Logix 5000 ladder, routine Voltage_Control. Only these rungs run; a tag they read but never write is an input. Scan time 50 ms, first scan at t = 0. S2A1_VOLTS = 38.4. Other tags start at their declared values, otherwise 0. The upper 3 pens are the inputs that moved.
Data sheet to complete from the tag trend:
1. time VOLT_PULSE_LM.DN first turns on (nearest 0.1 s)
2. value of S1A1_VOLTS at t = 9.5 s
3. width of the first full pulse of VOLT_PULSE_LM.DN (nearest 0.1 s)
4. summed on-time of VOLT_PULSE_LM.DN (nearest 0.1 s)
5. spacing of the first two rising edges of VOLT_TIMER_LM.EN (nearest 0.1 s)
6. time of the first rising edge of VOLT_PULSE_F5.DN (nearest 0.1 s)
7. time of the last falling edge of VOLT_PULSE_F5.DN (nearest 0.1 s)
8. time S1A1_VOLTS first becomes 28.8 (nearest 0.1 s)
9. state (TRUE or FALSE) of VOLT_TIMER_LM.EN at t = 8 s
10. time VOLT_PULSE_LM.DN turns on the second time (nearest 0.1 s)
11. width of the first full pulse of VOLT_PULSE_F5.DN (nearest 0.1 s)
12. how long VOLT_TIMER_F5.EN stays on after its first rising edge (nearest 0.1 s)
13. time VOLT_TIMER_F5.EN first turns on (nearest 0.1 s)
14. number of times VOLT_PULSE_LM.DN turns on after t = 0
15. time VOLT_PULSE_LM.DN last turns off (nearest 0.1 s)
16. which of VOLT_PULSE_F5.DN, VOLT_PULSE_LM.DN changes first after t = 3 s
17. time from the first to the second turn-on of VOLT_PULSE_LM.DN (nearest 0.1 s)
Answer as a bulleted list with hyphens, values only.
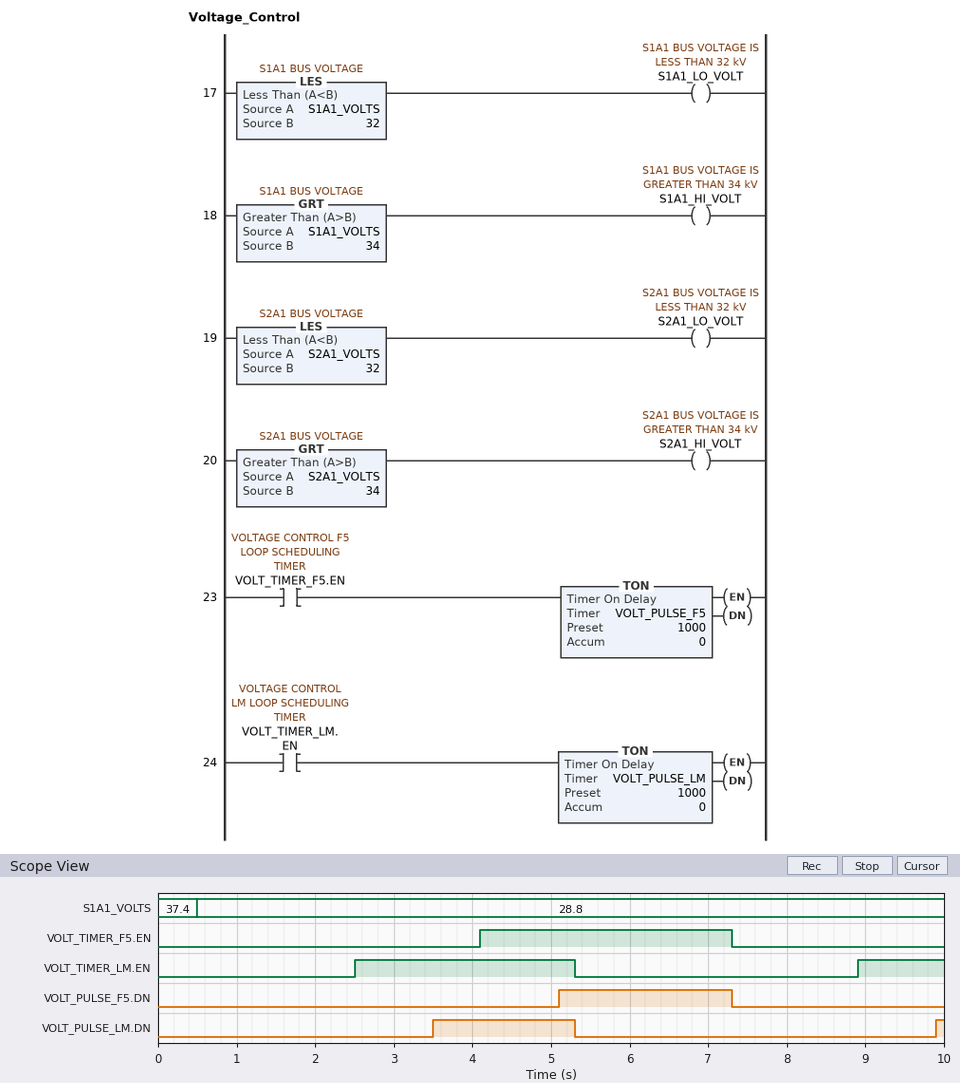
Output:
- 3.5 s
- 28.8
- 1.8 s
- 1.9 s
- 6.4 s
- 5.1 s
- 7.3 s
- 0.5 s
- FALSE
- 9.9 s
- 2.2 s
- 3.2 s
- 4.1 s
- 2
- 5.3 s
- VOLT_PULSE_LM.DN
- 6.4 s
